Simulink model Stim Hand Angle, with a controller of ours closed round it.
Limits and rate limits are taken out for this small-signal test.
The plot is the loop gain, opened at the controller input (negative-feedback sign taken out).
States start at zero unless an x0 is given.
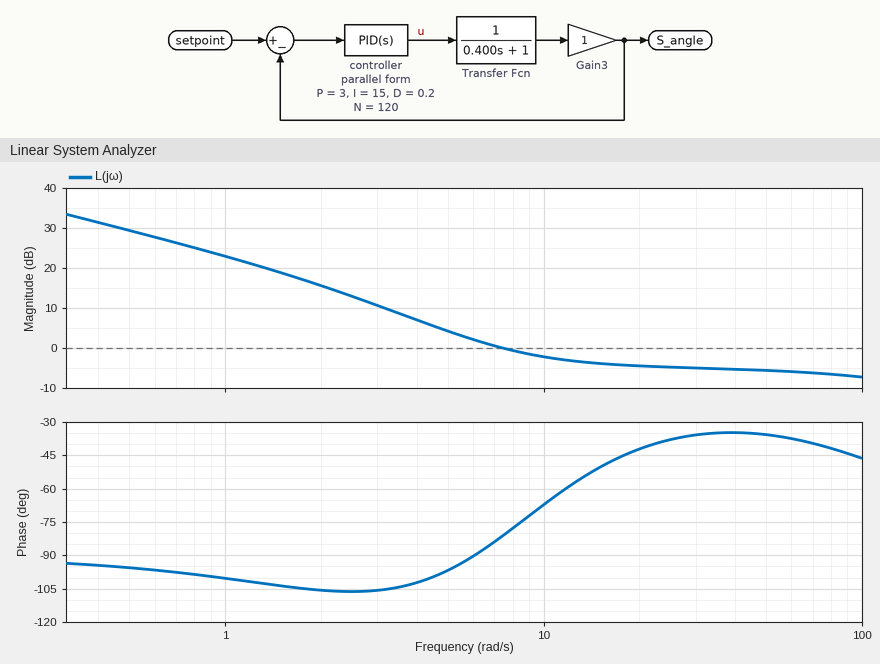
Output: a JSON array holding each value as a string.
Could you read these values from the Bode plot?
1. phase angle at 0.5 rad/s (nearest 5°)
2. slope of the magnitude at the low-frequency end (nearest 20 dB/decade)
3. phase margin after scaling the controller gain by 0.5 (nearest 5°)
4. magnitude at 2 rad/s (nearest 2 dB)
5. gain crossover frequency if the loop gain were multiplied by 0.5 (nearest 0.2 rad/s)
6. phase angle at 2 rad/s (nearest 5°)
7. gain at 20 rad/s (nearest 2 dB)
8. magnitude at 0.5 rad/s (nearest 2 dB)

["-95°", "-20 dB/decade", "80°", "16 dB", "4.4 rad/s", "-105°", "-4 dB", "30 dB"]
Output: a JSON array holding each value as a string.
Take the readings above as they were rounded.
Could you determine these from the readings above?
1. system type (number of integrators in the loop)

["1"]
